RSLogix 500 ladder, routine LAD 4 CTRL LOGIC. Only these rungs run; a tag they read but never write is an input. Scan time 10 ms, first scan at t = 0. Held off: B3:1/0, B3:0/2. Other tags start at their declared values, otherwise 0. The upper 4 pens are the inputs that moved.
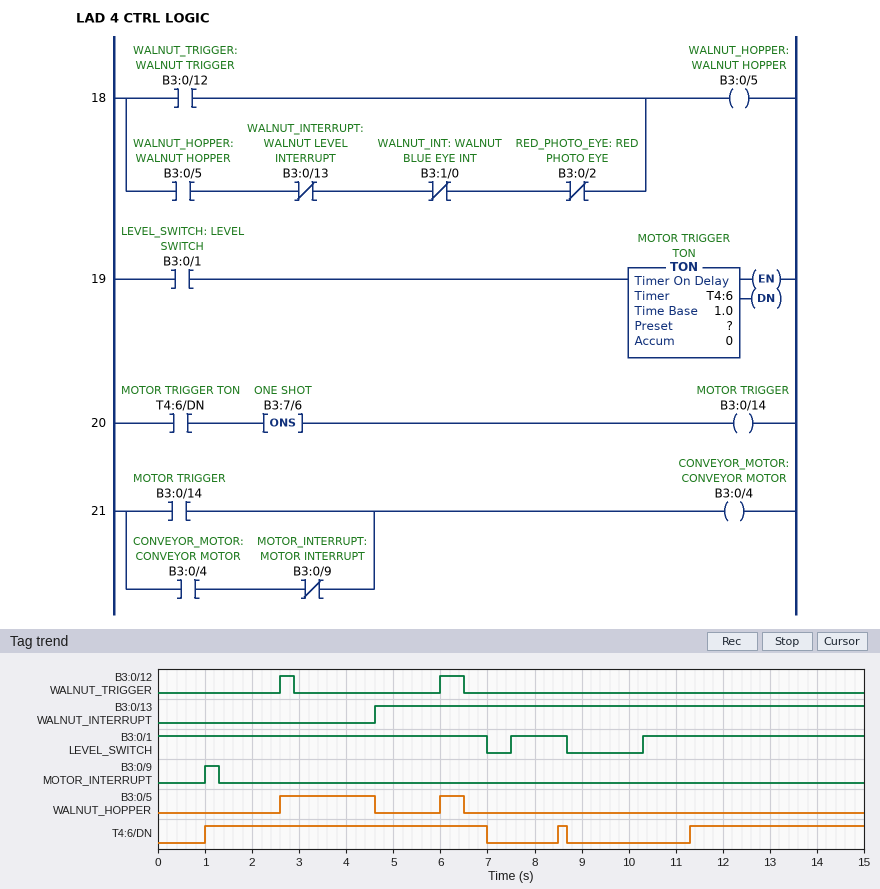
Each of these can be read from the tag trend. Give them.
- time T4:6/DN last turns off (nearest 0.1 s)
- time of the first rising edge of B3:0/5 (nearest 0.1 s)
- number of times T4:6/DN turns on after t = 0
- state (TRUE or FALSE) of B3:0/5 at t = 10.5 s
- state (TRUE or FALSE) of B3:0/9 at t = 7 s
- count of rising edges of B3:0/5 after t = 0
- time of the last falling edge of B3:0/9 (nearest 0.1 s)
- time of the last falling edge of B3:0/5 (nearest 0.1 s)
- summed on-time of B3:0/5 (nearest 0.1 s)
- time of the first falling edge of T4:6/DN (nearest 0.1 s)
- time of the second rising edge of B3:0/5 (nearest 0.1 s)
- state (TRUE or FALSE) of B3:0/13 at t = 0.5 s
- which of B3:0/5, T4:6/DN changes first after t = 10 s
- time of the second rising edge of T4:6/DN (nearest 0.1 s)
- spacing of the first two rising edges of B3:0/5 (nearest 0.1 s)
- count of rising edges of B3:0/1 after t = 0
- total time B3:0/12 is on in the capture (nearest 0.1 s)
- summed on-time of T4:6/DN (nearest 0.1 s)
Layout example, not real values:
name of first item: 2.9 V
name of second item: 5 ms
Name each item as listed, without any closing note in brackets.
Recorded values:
time T4:6/DN last turns off: 8.7 s
time of the first rising edge of B3:0/5: 2.6 s
number of times T4:6/DN turns on after t = 0: 3
state (TRUE or FALSE) of B3:0/5 at t = 10.5 s: FALSE
state (TRUE or FALSE) of B3:0/9 at t = 7 s: FALSE
count of rising edges of B3:0/5 after t = 0: 2
time of the last falling edge of B3:0/9: 1.3 s
time of the last falling edge of B3:0/5: 6.5 s
summed on-time of B3:0/5: 2.5 s
time of the first falling edge of T4:6/DN: 7.0 s
time of the second rising edge of B3:0/5: 6.0 s
state (TRUE or FALSE) of B3:0/13 at t = 0.5 s: FALSE
which of B3:0/5, T4:6/DN changes first after t = 10 s: T4:6/DN
time of the second rising edge of T4:6/DN: 8.5 s
spacing of the first two rising edges of B3:0/5: 3.4 s
count of rising edges of B3:0/1 after t = 0: 2
total time B3:0/12 is on in the capture: 0.8 s
summed on-time of T4:6/DN: 9.9 s
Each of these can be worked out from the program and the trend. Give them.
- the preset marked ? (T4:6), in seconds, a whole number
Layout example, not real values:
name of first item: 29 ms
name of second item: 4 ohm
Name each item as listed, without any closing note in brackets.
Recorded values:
the preset marked ? (T4:6), in seconds, a whole number: 1 s
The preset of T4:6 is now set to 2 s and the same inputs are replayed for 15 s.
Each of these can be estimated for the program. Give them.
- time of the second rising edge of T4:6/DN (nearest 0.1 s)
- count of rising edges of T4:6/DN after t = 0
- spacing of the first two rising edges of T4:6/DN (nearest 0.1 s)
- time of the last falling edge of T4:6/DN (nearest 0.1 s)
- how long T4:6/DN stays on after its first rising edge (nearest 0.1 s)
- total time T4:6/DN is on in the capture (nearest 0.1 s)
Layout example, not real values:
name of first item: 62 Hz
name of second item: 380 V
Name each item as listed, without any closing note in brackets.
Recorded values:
time of the second rising edge of T4:6/DN: 12.3 s
count of rising edges of T4:6/DN after t = 0: 2
spacing of the first two rising edges of T4:6/DN: 10.3 s
time of the last falling edge of T4:6/DN: 7.0 s
how long T4:6/DN stays on after its first rising edge: 5.0 s
total time T4:6/DN is on in the capture: 7.7 s
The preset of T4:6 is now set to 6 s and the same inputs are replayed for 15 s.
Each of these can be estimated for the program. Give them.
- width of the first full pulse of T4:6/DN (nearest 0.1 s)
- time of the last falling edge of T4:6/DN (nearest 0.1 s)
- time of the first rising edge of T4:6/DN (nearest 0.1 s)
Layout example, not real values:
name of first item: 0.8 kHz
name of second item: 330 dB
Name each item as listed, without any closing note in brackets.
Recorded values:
width of the first full pulse of T4:6/DN: 1.0 s
time of the last falling edge of T4:6/DN: 7.0 s
time of the first rising edge of T4:6/DN: 6.0 s
